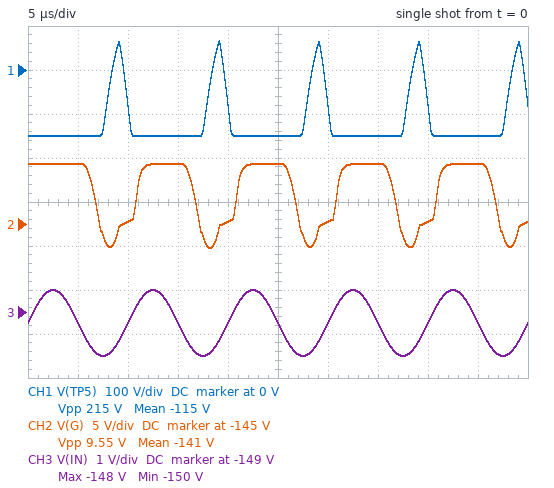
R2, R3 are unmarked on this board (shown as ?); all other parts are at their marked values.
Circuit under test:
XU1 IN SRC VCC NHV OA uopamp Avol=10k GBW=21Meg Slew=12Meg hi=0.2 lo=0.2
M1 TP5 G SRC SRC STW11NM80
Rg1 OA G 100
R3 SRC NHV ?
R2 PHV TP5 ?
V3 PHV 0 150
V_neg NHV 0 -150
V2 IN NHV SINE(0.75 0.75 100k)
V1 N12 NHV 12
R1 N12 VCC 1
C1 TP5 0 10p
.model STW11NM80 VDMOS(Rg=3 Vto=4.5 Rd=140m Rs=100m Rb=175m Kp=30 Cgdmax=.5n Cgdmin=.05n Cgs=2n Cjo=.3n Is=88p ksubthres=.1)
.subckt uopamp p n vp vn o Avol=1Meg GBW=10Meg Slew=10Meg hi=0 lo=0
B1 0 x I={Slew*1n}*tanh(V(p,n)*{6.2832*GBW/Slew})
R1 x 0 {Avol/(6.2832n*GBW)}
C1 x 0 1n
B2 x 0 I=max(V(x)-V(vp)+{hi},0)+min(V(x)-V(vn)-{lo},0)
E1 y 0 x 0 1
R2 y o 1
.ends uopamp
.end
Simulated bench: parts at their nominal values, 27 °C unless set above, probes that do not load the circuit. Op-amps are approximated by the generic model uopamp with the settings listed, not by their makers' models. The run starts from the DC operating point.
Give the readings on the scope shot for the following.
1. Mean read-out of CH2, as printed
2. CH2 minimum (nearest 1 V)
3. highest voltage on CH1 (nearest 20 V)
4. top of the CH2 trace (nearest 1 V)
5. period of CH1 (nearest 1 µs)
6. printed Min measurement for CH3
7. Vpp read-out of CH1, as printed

-141 V
-148 V
60 V
-138 V
10 µs
-150 V
215 V
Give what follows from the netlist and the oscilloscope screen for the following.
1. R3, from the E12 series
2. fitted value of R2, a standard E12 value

27 Ω
15 kΩ
